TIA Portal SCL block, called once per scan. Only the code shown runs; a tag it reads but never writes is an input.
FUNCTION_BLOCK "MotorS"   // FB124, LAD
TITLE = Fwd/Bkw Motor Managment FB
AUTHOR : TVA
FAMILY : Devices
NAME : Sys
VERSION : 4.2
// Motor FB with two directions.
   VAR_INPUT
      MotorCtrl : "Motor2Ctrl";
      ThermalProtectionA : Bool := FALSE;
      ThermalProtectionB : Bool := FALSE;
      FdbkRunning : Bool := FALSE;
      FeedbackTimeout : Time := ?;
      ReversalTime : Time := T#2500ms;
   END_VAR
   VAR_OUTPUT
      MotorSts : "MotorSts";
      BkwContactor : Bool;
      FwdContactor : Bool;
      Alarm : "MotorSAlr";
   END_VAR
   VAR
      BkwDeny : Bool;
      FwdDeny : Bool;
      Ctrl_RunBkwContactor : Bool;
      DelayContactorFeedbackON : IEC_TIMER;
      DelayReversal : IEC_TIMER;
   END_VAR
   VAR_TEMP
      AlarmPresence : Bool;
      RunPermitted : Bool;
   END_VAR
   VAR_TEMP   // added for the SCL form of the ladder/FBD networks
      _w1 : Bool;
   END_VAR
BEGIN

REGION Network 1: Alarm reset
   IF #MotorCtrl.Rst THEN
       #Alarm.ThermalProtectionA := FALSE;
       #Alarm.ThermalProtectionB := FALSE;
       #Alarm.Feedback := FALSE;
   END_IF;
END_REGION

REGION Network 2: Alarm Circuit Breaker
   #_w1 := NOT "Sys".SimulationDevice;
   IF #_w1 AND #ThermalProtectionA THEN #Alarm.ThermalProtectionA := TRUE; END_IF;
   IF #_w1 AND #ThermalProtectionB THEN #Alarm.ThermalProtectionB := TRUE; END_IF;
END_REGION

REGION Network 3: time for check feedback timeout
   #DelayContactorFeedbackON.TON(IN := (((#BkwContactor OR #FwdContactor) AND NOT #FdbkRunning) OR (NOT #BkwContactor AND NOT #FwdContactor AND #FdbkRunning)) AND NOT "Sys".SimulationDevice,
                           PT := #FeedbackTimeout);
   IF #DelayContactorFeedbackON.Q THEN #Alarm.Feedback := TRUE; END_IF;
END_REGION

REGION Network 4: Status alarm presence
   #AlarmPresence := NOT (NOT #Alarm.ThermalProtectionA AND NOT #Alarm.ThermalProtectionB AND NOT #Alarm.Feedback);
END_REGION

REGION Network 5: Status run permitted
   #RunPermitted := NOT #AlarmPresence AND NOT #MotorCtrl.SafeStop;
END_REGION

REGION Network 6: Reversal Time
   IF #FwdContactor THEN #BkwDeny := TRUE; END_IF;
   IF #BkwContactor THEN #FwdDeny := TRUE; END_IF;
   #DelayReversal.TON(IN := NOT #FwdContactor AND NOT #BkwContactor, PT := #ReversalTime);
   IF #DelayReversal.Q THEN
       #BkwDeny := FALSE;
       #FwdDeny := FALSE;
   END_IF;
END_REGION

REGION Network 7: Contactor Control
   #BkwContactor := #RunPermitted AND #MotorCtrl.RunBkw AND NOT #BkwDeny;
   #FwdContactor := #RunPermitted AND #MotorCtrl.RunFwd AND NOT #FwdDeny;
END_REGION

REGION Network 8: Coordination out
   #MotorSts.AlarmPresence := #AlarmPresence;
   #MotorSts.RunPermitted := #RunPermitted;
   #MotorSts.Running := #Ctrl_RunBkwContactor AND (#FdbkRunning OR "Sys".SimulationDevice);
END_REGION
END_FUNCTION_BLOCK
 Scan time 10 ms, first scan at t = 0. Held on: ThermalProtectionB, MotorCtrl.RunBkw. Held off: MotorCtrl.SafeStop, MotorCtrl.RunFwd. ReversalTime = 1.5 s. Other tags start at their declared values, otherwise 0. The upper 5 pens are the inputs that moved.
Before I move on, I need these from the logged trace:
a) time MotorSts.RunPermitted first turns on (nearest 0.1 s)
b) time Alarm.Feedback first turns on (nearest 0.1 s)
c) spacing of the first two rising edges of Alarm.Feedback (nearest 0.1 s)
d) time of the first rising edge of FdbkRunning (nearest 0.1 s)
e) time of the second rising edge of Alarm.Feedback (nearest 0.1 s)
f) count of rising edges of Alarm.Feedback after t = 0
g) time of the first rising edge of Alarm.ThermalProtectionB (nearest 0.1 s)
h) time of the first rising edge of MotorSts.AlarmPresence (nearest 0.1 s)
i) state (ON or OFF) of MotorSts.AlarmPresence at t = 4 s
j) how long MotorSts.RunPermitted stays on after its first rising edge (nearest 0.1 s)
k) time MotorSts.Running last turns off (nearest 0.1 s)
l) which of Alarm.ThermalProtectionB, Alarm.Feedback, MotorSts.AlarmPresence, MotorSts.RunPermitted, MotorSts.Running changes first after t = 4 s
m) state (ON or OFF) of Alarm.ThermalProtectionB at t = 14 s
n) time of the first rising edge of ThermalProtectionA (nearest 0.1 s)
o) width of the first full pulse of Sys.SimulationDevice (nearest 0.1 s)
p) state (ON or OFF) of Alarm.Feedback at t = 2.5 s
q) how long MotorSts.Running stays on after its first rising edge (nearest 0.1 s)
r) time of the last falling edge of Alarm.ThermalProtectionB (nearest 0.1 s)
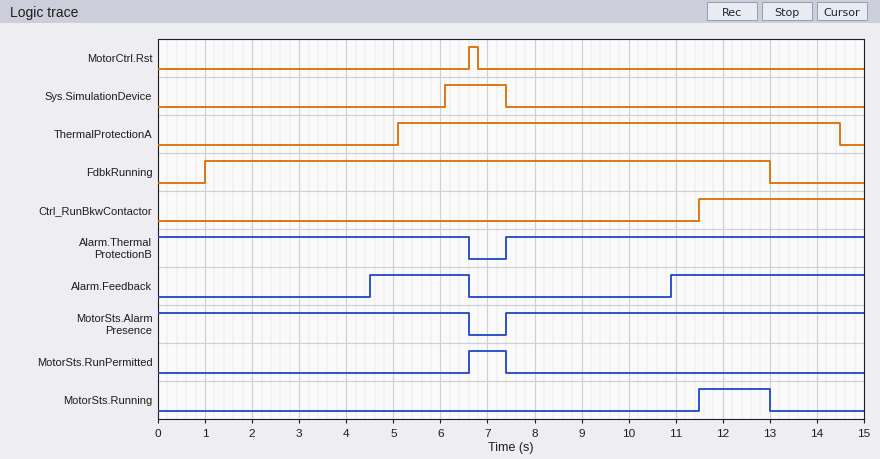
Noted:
6.6 s
4.5 s
6.4 s
1.0 s
10.9 s
2
7.4 s
7.4 s
ON
0.8 s
13.0 s
Alarm.Feedback
ON
5.1 s
1.3 s
OFF
1.5 s
6.6 s
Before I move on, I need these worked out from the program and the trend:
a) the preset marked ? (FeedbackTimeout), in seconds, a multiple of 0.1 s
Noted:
3.5 s
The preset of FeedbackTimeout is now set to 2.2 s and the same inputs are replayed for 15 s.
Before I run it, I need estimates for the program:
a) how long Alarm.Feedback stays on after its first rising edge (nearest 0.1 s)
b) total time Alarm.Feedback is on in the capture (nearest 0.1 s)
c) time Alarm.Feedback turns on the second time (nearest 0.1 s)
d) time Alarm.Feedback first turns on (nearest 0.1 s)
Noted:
3.4 s
8.8 s
9.6 s
3.2 s
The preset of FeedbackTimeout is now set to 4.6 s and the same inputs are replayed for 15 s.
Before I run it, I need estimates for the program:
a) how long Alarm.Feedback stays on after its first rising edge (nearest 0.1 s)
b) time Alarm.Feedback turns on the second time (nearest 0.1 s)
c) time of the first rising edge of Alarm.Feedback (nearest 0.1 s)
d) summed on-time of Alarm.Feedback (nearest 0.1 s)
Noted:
1.0 s
12.0 s
5.6 s
4.0 s
